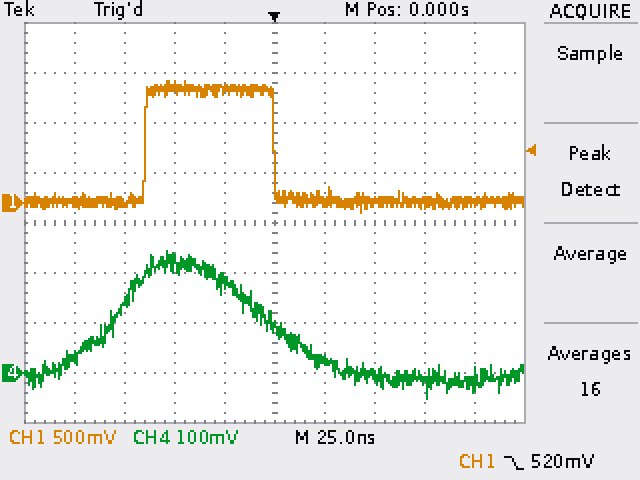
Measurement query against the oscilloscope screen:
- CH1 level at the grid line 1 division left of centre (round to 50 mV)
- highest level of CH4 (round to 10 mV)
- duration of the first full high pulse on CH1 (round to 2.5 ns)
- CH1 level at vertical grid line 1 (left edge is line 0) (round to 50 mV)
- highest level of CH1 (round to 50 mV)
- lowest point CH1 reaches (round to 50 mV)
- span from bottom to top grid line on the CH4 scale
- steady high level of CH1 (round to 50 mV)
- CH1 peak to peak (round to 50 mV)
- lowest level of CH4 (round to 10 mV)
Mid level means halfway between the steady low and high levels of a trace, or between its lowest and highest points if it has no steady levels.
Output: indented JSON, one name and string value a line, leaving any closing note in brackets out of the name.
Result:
{
  "CH1 level at the grid line 1 division left of centre": "1.15 V",
  "highest level of CH4": "240 mV",
  "duration of the first full high pulse on CH1": "65.0 ns",
  "CH1 level at vertical grid line 1 (left edge is line 0)": "0 mV",
  "highest level of CH1": "1.20 V",
  "lowest point CH1 reaches": "-100 mV",
  "span from bottom to top grid line on the CH4 scale": "800 mV",
  "steady high level of CH1": "1.15 V",
  "CH1 peak to peak": "1.30 V",
  "lowest level of CH4": "-50 mV"
}
